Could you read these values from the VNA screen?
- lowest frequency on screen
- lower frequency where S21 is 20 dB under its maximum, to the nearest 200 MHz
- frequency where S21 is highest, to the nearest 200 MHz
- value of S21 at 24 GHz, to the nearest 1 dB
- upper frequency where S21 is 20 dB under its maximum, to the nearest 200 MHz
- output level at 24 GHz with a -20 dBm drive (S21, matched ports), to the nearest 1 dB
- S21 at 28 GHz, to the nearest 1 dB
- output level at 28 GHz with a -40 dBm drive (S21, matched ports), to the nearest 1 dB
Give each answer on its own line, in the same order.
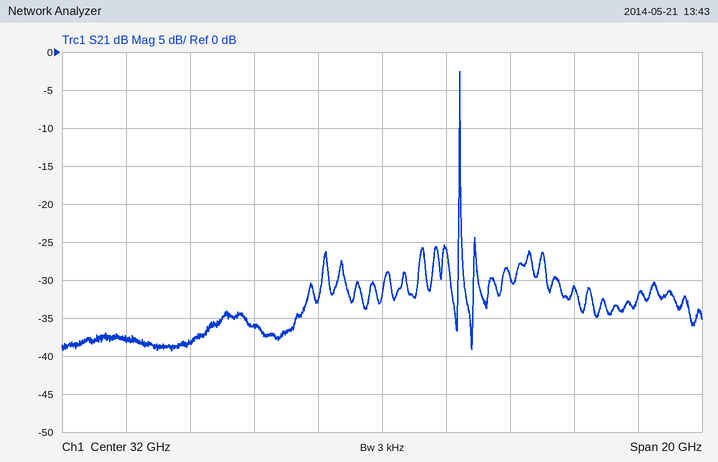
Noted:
22 GHz
34.4 GHz
34.4 GHz
-38 dB
34.4 GHz
-58 dBm
-36 dB
-76 dBm
